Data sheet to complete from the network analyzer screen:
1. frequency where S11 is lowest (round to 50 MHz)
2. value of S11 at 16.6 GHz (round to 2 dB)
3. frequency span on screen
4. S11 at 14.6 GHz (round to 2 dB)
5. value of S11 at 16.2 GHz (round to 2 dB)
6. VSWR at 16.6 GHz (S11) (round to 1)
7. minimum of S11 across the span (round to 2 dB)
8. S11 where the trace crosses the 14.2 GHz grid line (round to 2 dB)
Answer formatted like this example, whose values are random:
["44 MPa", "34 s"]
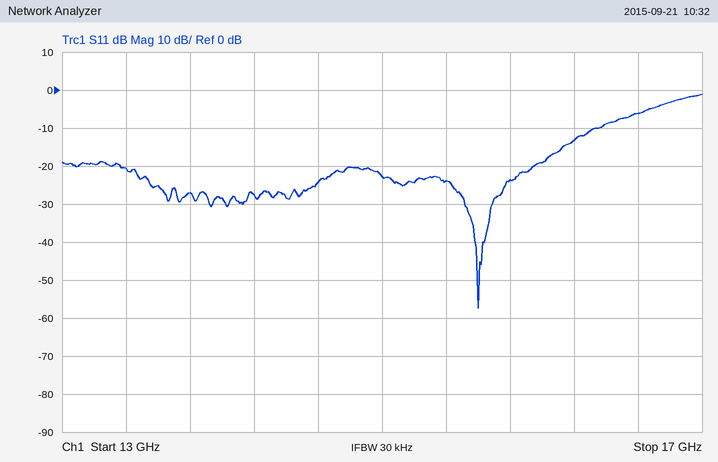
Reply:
["15.60 GHz", "-6 dB", "4 GHz", "-24 dB", "-14 dB", "3", "-58 dB", "-28 dB"]
